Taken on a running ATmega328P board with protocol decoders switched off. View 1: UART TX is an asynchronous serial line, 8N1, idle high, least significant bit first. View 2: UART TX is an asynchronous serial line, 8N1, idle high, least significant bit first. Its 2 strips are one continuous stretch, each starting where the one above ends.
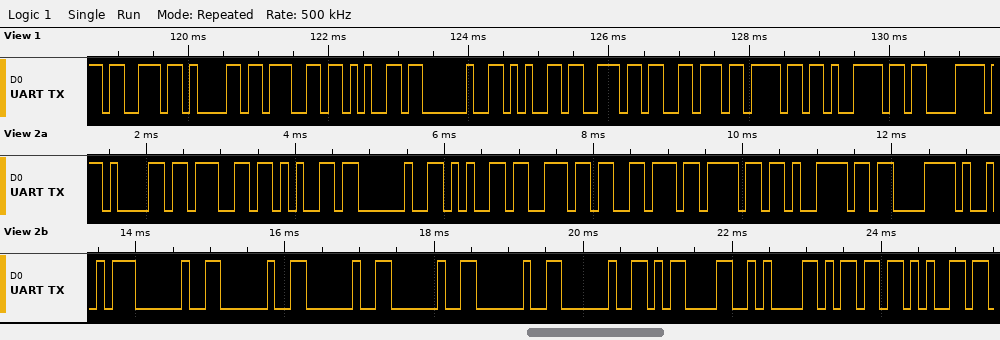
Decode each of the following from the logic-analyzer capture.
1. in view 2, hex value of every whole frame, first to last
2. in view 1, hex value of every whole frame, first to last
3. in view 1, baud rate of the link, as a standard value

61 67 65 20 65 6E 76 6F 79 C3 A9 20 20 20 20 20 20 0D 0A 6D 65
0x73 0x61 0x67 0x65 0x20 0x65 0x6E 0x76 0x6F 0x79 0xC3
9600 baud
